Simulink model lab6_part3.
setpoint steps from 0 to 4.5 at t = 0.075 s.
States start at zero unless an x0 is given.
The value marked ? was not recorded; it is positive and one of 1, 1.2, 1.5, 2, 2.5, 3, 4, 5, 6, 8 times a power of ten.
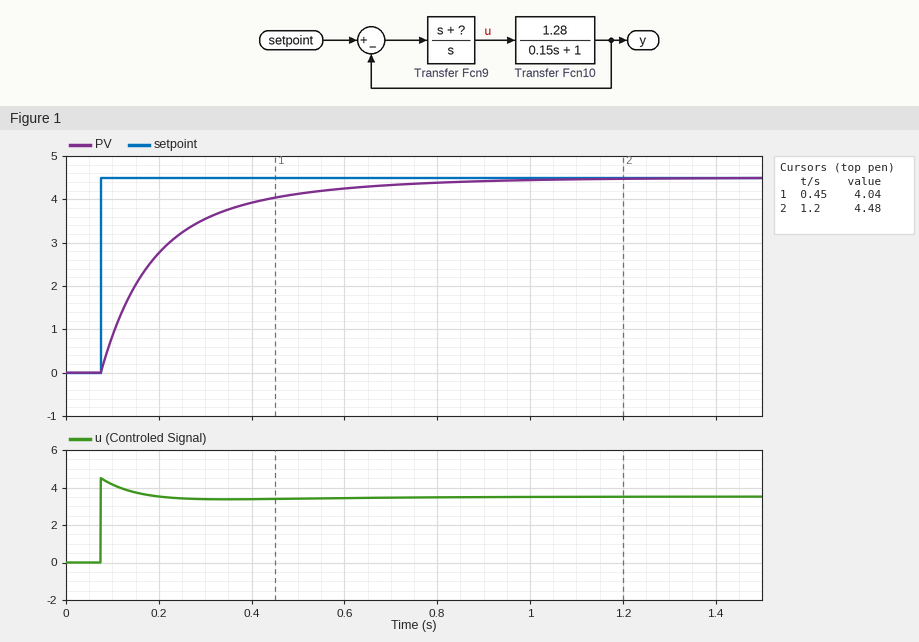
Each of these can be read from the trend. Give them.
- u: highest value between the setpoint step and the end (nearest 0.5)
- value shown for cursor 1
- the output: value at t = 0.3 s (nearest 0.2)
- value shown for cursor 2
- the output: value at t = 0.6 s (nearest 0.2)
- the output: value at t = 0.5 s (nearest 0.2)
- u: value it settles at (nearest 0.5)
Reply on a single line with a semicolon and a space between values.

4.5; 4.04; 3.6; 4.48; 4.2; 4.2; 3.5
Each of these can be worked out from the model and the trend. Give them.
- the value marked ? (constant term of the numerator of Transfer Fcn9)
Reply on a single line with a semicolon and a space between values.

5
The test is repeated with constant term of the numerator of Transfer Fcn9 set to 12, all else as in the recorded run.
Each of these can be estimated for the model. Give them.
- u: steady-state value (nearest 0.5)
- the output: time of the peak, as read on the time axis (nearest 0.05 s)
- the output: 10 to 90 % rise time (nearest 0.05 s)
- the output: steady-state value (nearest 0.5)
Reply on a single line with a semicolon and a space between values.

3.5; 0.40 s; 0.15 s; 4.5
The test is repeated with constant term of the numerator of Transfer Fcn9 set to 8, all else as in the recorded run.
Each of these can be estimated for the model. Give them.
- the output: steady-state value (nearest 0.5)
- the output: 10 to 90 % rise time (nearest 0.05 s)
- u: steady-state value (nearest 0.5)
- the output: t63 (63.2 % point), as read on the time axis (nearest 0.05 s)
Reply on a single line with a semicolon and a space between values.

4.5; 0.20 s; 3.5; 0.20 s
